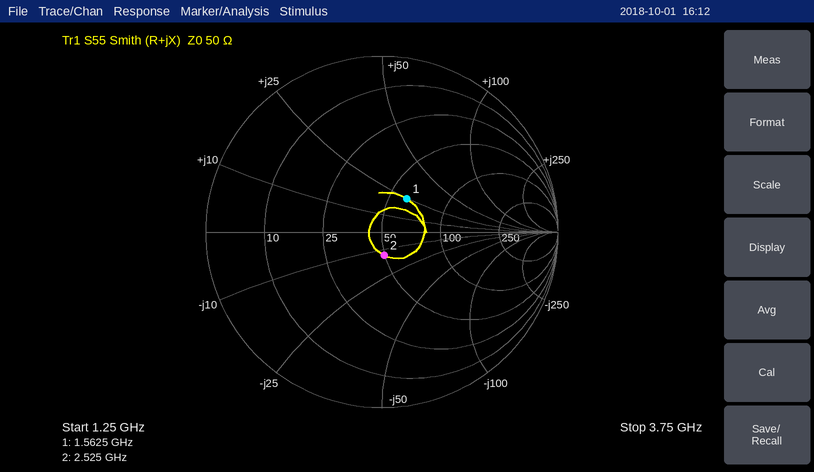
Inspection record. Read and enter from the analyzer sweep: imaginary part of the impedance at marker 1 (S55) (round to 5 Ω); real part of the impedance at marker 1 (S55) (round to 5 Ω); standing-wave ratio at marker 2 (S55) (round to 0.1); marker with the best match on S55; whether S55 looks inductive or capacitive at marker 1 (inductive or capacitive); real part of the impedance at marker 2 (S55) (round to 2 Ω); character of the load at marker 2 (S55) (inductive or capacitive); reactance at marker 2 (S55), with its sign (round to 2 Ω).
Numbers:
+25 Ω
60 Ω
1.3
marker 2
inductive
50 Ω
capacitive
-14 Ω
